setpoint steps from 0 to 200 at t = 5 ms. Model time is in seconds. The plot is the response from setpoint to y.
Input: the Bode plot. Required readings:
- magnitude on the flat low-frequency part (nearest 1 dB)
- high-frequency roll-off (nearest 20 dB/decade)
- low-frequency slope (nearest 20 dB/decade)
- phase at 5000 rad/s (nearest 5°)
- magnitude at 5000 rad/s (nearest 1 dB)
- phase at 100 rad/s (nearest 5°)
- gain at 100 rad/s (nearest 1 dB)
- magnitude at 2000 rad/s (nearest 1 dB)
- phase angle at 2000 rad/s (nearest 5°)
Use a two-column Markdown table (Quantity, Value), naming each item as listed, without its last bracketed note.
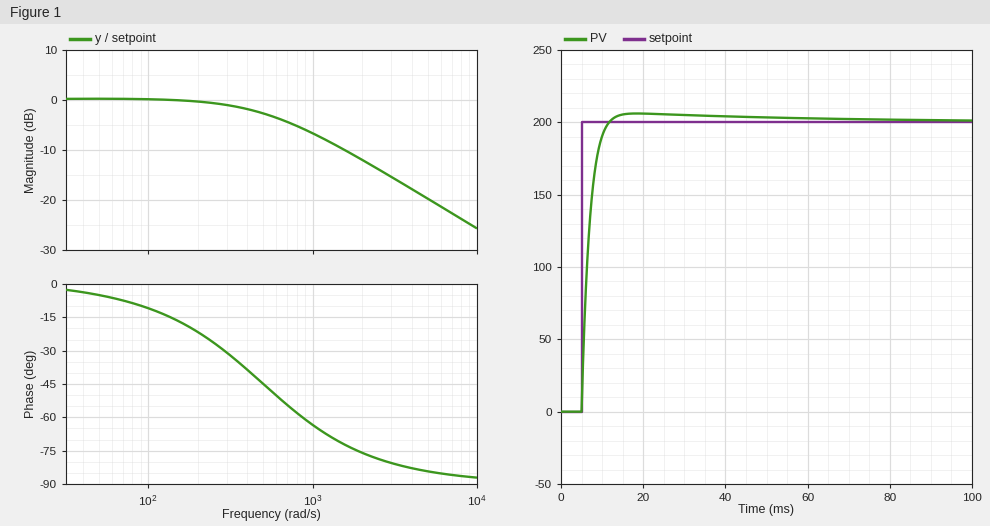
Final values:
| Quantity | Value |
|---|---|
| magnitude on the flat low-frequency part | 0 dB |
| high-frequency roll-off | -20 dB/decade |
| low-frequency slope | 0 dB/decade |
| phase at 5000 rad/s | -85° |
| magnitude at 5000 rad/s | -20 dB |
| phase at 100 rad/s | -10° |
| gain at 100 rad/s | 0 dB |
| magnitude at 2000 rad/s | -12 dB |
| phase angle at 2000 rad/s | -75° |
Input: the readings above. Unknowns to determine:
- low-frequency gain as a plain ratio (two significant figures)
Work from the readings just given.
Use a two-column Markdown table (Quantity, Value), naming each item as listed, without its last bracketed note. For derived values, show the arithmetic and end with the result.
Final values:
| Quantity | Value |
|---|---|
| low-frequency gain as a plain ratio | 10^(0 / 20) = 1.0 |
